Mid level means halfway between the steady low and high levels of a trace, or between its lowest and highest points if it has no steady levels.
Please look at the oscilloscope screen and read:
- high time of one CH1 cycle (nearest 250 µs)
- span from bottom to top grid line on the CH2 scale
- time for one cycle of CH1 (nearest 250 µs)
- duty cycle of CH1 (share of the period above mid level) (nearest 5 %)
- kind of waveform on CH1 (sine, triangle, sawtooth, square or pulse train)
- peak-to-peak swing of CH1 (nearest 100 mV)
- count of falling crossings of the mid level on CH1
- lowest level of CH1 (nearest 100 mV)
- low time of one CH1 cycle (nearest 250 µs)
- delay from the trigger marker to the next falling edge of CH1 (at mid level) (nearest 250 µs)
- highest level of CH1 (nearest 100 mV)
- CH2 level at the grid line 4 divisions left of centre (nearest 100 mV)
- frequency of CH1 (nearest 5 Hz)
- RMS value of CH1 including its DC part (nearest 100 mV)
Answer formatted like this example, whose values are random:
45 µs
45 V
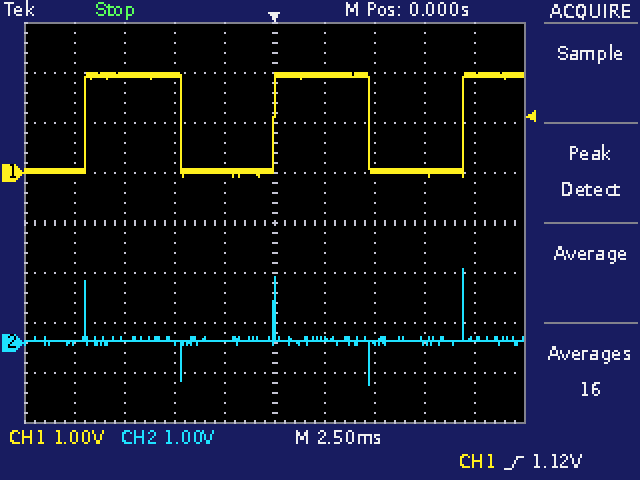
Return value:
4.75 ms
8 V
9.50 ms
50 %
square
2.1 V
2
-100 mV
4.75 ms
4.75 ms
2.0 V
0.0 V
105 Hz
1.4 V
